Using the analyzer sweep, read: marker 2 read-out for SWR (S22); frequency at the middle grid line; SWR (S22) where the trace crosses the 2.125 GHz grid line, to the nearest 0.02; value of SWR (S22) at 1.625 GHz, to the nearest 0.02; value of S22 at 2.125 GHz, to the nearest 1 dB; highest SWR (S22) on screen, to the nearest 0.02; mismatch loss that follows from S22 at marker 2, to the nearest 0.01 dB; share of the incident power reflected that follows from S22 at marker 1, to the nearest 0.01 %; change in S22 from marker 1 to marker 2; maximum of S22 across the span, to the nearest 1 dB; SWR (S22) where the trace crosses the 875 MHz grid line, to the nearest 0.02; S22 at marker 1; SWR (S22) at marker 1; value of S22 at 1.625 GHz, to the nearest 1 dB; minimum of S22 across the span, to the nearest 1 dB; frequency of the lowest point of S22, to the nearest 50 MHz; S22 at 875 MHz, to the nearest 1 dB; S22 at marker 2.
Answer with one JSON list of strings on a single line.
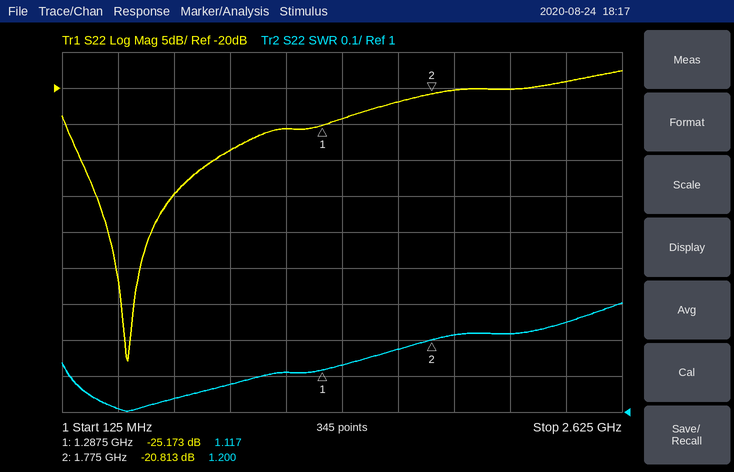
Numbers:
["1.200", "1.375 GHz", "1.22", "1.18", "-20 dB", "1.30", "0.04 dB", "0.30 %", "4.360 dB", "-18 dB", "1.08", "-25.173 dB", "1.117", "-22 dB", "-58 dB", "400 MHz", "-29 dB", "-20.813 dB"]
